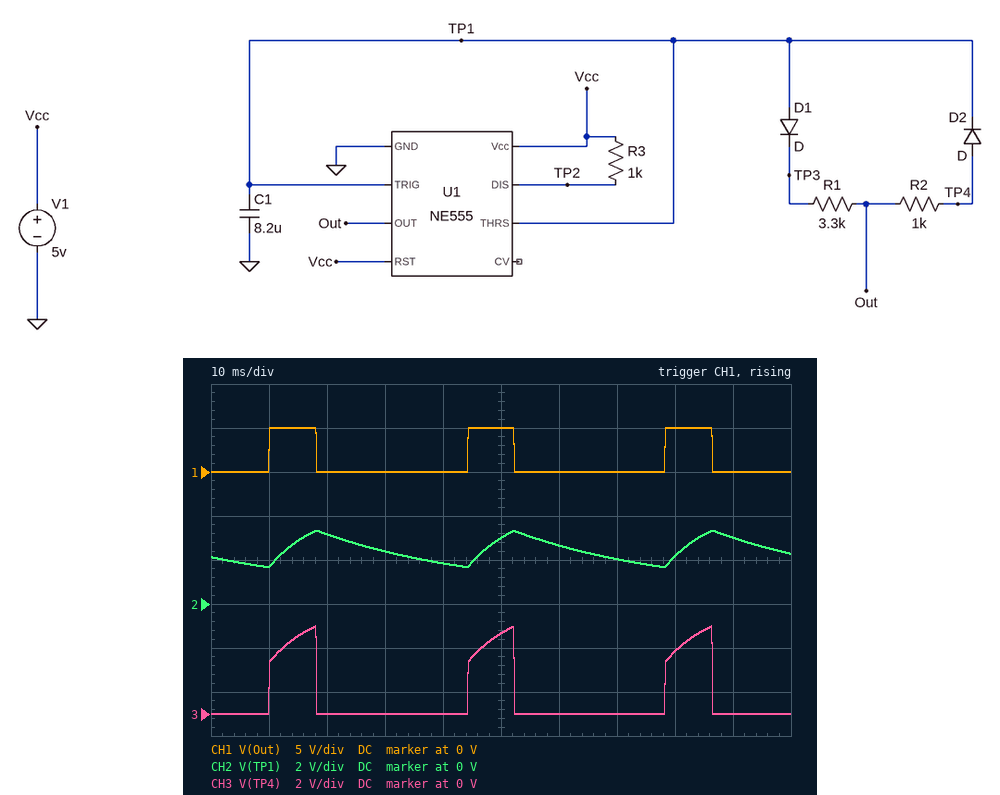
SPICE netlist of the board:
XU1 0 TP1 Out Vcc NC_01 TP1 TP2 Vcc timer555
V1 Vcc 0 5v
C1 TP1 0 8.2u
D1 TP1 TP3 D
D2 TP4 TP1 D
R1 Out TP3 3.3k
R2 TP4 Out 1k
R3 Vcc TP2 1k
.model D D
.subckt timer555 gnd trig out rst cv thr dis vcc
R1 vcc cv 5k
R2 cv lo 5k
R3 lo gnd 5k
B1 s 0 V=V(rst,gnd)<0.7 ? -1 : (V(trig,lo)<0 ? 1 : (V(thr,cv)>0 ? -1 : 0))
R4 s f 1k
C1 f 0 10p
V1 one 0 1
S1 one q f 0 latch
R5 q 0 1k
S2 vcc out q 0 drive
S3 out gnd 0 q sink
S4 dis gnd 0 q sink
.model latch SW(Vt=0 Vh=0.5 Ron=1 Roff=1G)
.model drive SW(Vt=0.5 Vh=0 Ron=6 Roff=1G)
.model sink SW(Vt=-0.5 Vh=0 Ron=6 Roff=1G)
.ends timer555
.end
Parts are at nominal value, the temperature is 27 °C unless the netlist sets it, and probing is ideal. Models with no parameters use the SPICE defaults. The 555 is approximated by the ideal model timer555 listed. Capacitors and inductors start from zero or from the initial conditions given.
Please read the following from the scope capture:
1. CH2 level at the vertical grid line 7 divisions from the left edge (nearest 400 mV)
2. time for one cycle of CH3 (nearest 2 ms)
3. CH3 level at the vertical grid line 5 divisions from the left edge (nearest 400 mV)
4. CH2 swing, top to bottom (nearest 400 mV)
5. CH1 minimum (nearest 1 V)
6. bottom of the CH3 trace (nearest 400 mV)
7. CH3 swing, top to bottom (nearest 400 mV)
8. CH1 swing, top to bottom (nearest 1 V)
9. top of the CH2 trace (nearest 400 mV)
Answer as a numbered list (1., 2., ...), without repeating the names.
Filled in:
1. 2.0 V
2. 34 ms
3. 3.6 V
4. 1.6 V
5. 0 V
6. 0 V
7. 4.0 V
8. 5 V
9. 3.2 V
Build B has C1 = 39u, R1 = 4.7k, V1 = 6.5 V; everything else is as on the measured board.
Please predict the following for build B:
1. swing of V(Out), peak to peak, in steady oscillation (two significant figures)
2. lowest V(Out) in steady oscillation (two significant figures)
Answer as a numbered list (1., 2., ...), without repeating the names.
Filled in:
1. 6.5 V
2. 2.0 mV
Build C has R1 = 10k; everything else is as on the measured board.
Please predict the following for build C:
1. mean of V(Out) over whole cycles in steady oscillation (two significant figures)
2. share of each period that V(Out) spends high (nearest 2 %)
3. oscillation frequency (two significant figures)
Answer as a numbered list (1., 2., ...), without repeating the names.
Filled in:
1. 470 mV
2. 10 %
3. 12 Hz
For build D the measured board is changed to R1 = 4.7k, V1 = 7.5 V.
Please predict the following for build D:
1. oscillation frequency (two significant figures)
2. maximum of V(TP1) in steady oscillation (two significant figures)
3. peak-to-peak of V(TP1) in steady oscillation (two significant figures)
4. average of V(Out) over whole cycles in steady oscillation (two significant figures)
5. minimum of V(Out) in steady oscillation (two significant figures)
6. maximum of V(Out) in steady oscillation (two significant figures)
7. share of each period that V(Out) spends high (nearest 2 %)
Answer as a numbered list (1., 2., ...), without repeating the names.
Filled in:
1. 25 Hz
2. 5.0 V
3. 2.5 V
4. 1.3 V
5. 2.4 mV
6. 7.5 V
7. 18 %
